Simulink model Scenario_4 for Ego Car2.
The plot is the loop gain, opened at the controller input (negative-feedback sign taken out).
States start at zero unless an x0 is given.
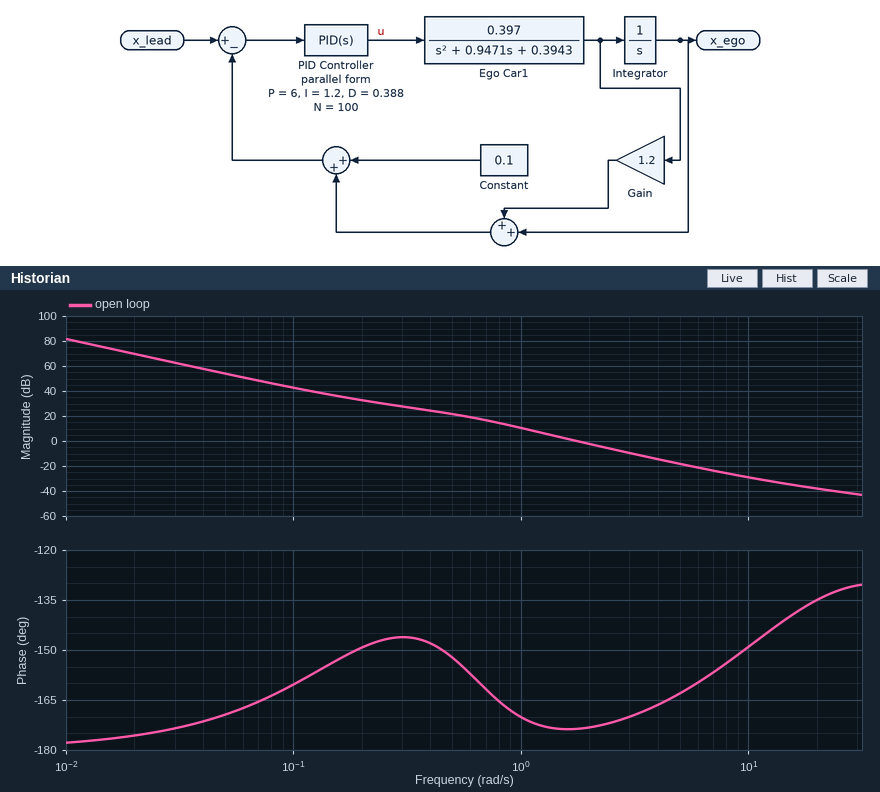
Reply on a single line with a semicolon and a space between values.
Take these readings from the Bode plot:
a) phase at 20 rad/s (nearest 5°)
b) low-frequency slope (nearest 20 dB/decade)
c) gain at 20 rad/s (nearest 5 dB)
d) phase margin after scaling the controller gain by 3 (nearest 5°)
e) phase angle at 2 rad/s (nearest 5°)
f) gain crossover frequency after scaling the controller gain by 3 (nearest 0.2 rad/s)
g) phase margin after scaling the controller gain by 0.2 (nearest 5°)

-135°; -40 dB/decade; -40 dB; 10°; -175°; 3.0 rad/s; 15°
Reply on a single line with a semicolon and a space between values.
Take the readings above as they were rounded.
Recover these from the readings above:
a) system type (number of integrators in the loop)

2
